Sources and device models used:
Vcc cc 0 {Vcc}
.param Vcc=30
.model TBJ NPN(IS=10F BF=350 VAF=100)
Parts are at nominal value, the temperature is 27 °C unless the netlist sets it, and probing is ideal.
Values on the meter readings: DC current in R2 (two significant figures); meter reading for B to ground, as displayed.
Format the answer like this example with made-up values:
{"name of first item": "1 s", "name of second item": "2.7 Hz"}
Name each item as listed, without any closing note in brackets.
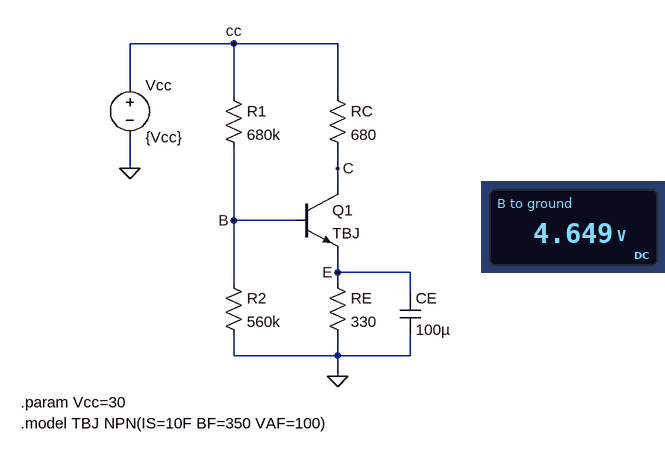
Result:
{"DC current in R2": "8.3 µA", "meter reading for B to ground, as displayed": "4.649 V"}
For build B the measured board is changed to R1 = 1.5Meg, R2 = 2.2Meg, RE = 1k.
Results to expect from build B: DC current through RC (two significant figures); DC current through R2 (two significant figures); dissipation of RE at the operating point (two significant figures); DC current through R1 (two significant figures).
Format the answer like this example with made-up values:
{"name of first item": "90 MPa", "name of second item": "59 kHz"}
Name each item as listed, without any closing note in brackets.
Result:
{"DC current through RC": "5.5 mA", "DC current through R2": "2.8 µA", "dissipation of RE at the operating point": "30 mW", "DC current through R1": "16 µA"}
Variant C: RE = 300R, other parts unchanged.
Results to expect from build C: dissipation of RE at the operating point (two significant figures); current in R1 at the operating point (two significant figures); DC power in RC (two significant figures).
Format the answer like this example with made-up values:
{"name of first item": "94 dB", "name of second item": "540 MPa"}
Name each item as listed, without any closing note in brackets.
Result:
{"dissipation of RE at the operating point": "45 mW", "current in R1 at the operating point": "38 µA", "DC power in RC": "100 mW"}
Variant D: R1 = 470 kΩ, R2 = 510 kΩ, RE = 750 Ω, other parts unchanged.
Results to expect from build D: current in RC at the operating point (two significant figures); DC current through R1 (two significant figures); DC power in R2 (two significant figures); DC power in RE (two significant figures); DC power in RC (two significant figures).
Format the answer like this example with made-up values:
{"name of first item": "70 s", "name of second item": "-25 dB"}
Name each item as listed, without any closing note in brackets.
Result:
{"current in RC at the operating point": "11 mA", "DC current through R1": "45 µA", "DC power in R2": "160 µW", "DC power in RE": "90 mW", "DC power in RC": "81 mW"}
